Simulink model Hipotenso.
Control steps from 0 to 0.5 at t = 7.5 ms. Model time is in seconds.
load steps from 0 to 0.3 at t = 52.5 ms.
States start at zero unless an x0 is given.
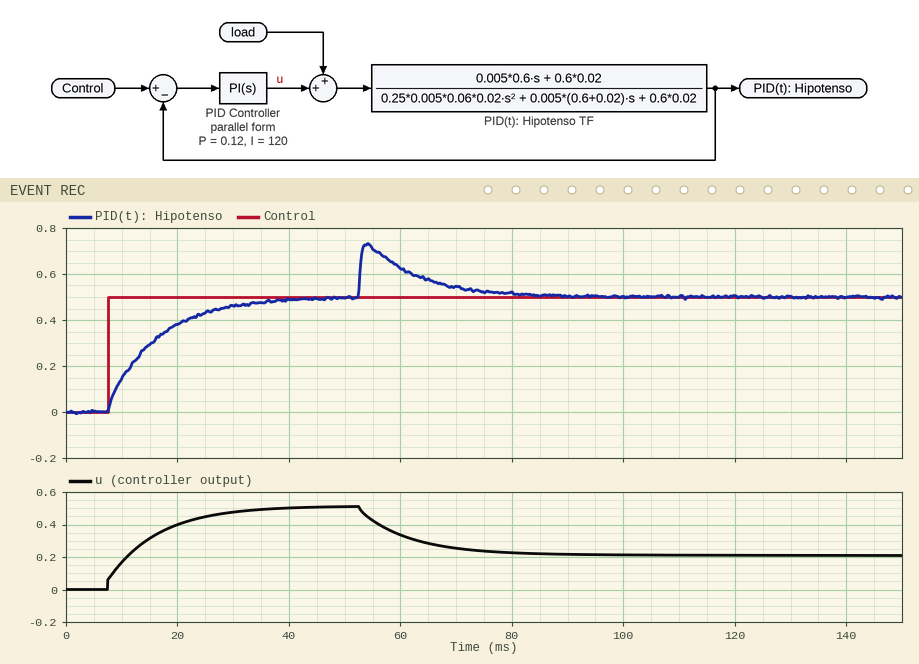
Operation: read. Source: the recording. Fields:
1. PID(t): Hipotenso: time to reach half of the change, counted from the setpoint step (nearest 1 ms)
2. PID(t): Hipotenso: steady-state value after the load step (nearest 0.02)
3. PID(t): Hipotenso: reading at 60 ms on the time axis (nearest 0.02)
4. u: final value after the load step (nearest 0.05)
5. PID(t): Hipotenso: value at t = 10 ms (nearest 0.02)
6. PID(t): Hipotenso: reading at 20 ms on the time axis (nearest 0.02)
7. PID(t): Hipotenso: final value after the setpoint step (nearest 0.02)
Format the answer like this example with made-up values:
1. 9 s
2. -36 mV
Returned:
1. 6 ms
2. 0.50
3. 0.62
4. 0.20
5. 0.14
6. 0.38
7. 0.50
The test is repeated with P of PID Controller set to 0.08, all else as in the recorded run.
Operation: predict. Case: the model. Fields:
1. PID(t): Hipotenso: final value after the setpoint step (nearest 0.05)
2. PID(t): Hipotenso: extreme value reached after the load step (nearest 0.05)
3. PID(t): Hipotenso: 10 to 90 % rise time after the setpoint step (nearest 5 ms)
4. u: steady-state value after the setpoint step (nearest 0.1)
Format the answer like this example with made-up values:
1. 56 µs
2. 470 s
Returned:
1. 0.50
2. 0.75
3. 20 ms
4. 0.5
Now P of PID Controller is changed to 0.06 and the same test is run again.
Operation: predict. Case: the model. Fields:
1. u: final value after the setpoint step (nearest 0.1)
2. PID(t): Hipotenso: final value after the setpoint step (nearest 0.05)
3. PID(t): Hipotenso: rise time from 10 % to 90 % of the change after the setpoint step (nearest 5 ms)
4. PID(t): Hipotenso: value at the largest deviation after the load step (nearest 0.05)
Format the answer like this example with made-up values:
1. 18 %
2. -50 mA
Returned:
1. 0.5
2. 0.50
3. 20 ms
4. 0.75
